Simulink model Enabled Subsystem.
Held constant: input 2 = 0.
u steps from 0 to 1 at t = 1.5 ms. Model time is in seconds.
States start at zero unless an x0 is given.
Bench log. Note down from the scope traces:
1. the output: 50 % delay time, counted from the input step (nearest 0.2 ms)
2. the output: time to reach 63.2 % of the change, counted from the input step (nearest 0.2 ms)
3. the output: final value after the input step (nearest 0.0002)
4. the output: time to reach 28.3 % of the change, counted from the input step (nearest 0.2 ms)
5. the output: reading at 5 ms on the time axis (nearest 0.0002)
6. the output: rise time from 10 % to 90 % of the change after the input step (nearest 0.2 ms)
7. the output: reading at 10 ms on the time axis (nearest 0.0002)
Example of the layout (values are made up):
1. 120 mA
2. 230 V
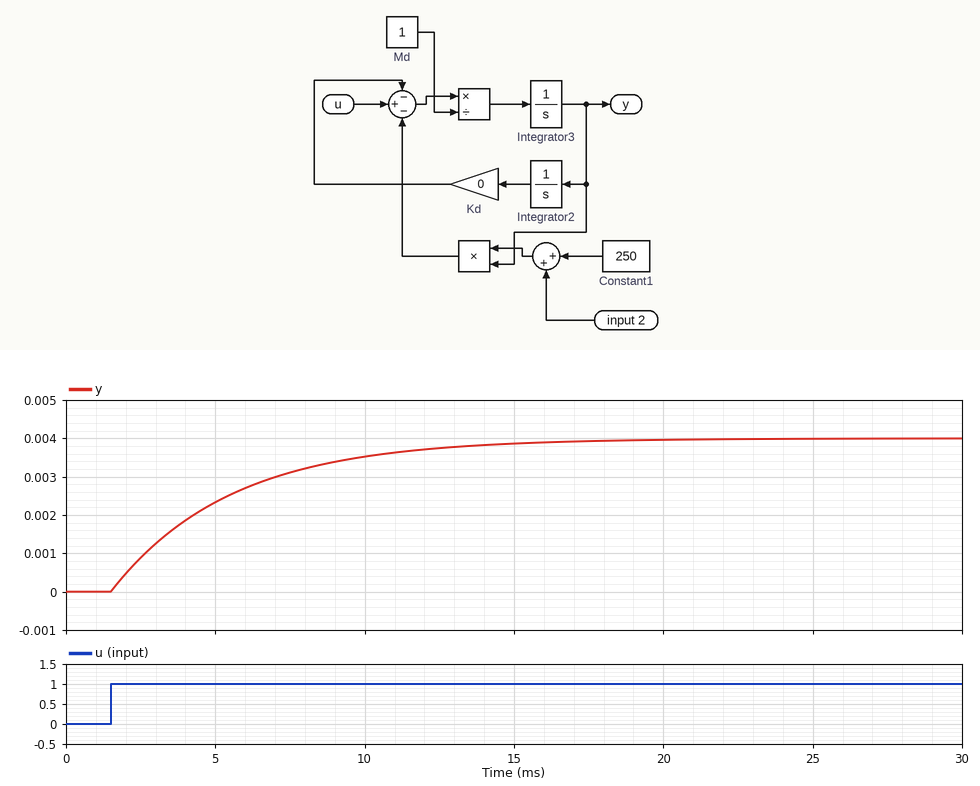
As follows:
1. 2.8 ms
2. 4.0 ms
3. 0.0040
4. 1.4 ms
5. 0.0024
6. 8.8 ms
7. 0.0036
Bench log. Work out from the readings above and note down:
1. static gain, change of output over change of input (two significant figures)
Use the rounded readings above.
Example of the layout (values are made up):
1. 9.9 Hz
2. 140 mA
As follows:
1. 0.0040
